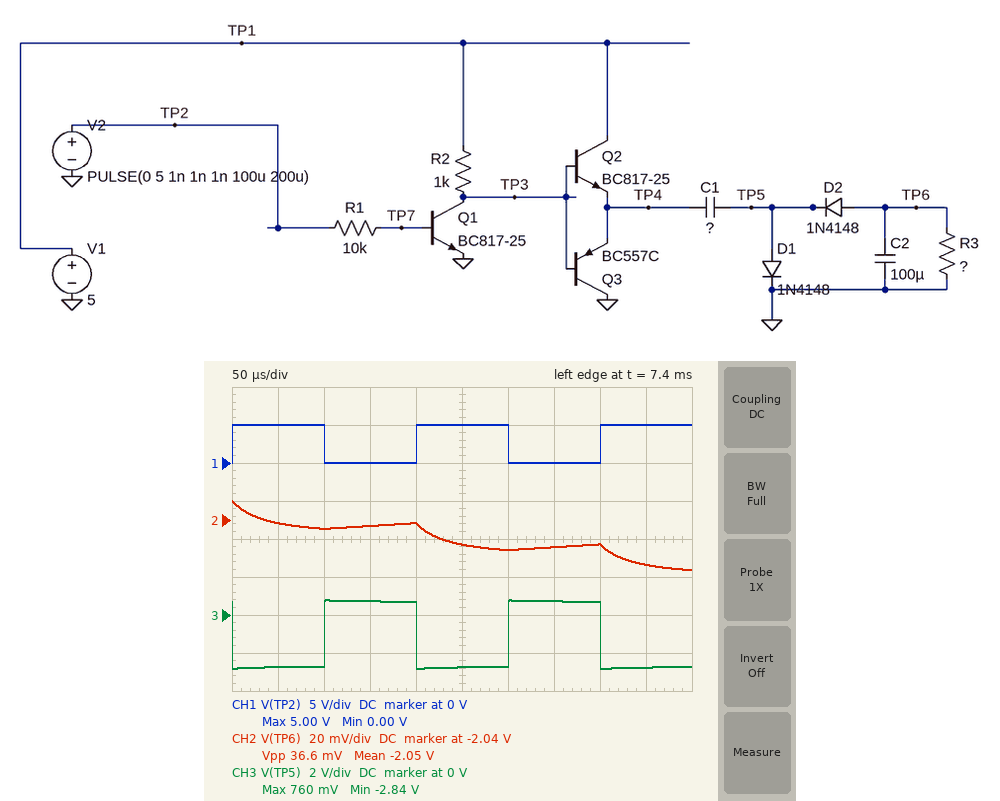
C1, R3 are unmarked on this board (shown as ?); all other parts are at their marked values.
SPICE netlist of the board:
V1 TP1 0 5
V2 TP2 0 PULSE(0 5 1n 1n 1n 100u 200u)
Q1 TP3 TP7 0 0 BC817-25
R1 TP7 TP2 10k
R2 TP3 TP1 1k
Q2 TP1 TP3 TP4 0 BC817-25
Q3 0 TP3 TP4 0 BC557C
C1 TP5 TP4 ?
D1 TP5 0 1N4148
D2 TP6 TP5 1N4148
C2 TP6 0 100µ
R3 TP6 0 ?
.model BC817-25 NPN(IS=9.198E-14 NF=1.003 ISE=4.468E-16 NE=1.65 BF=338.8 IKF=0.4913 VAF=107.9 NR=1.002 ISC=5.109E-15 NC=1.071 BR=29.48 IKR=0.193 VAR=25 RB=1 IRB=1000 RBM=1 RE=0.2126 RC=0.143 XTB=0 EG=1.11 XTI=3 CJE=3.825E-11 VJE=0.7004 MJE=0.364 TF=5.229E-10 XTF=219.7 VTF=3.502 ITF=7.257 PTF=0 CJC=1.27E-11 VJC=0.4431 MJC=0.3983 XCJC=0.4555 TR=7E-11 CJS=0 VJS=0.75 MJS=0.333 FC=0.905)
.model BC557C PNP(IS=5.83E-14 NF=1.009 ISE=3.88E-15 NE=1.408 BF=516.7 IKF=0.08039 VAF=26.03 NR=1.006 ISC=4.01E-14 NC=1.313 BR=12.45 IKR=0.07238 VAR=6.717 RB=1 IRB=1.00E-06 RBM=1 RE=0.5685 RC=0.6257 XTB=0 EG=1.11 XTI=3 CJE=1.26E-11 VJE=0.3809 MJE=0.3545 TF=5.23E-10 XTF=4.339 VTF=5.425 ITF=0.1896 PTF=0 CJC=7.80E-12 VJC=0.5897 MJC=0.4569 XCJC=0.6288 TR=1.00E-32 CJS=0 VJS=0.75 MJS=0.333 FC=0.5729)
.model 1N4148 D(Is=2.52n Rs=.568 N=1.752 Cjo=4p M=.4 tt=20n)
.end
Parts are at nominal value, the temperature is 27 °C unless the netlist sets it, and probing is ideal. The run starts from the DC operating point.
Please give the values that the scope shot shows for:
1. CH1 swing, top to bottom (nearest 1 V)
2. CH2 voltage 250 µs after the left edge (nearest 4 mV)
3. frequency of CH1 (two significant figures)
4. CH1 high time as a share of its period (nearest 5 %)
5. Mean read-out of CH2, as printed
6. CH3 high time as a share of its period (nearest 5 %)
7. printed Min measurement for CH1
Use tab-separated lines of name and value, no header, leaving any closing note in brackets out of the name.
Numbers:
CH1 swing, top to bottom	5 V
CH2 voltage 250 µs after the left edge	-2.052 V
frequency of CH1	5.0 kHz
CH1 high time as a share of its period	50 %
Mean read-out of CH2, as printed	-2.05 V
CH3 high time as a share of its period	50 %
printed Min measurement for CH1	0.00 V
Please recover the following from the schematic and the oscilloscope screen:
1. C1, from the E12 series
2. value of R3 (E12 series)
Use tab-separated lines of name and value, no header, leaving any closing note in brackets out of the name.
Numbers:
C1, from the E12 series	8.2 µF
value of R3	680 Ω
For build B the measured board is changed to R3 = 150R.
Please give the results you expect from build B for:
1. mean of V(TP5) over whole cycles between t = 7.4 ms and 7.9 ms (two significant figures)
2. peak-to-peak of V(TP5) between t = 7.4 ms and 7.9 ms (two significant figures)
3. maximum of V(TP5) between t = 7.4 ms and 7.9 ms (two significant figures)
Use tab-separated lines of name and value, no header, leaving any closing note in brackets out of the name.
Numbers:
mean of V(TP5) over whole cycles between t = 7.4 ms and 7.9 ms	-910 mV
peak-to-peak of V(TP5) between t = 7.4 ms and 7.9 ms	3.5 V
maximum of V(TP5) between t = 7.4 ms and 7.9 ms	820 mV
